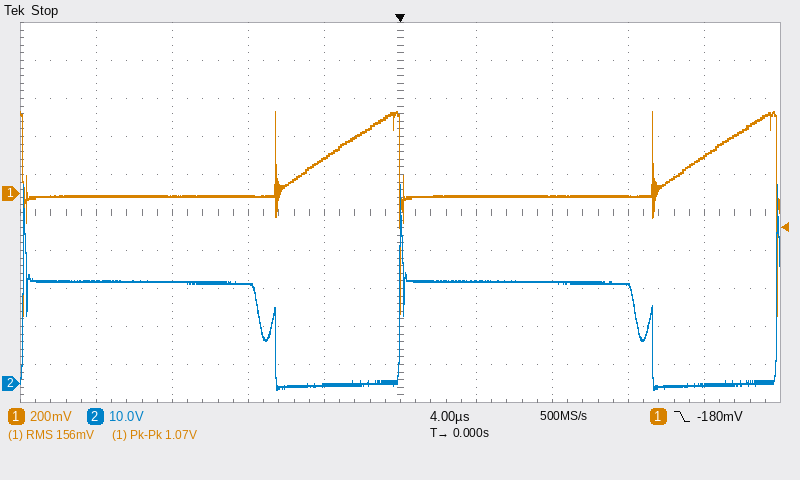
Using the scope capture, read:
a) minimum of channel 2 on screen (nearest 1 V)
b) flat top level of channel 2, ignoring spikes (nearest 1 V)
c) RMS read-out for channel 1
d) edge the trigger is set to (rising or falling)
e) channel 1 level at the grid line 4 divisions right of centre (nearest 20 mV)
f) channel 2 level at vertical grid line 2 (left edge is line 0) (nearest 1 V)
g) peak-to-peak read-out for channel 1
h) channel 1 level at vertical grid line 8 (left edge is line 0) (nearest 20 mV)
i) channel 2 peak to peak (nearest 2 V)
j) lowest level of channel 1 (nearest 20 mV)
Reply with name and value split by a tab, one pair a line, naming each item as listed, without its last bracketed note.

minimum of channel 2 on screen	-2 V
flat top level of channel 2, ignoring spikes	27 V
RMS read-out for channel 1	156 mV
edge the trigger is set to	falling
channel 1 level at the grid line 4 divisions right of centre	200 mV
channel 2 level at vertical grid line 2 (left edge is line 0)	27 V
peak-to-peak read-out for channel 1	1.07 V
channel 1 level at vertical grid line 8 (left edge is line 0)	-20 mV
channel 2 peak to peak	54 V
lowest level of channel 1	-640 mV
